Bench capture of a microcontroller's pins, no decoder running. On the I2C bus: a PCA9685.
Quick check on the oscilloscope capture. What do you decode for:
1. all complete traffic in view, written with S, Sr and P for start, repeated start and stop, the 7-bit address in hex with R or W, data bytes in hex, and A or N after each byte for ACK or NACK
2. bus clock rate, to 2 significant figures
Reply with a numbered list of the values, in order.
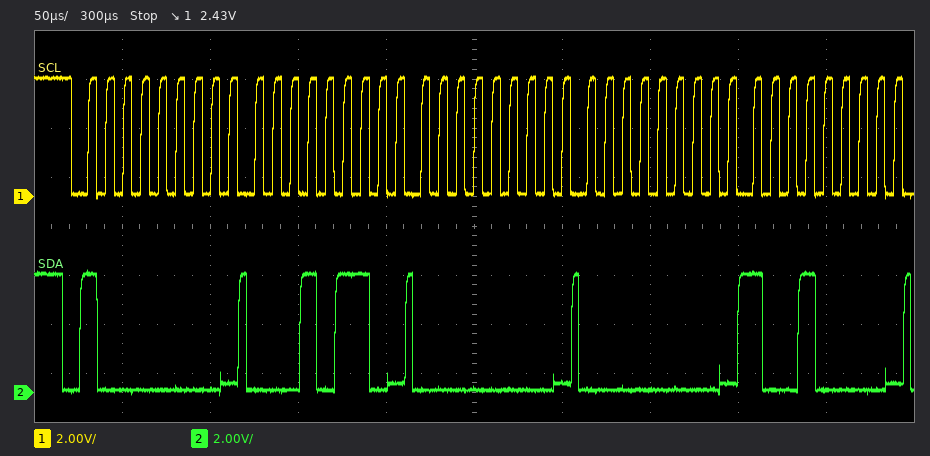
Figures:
1. S 40W A 16 A 00 A 00 A 90 A
2. 100 kHz
